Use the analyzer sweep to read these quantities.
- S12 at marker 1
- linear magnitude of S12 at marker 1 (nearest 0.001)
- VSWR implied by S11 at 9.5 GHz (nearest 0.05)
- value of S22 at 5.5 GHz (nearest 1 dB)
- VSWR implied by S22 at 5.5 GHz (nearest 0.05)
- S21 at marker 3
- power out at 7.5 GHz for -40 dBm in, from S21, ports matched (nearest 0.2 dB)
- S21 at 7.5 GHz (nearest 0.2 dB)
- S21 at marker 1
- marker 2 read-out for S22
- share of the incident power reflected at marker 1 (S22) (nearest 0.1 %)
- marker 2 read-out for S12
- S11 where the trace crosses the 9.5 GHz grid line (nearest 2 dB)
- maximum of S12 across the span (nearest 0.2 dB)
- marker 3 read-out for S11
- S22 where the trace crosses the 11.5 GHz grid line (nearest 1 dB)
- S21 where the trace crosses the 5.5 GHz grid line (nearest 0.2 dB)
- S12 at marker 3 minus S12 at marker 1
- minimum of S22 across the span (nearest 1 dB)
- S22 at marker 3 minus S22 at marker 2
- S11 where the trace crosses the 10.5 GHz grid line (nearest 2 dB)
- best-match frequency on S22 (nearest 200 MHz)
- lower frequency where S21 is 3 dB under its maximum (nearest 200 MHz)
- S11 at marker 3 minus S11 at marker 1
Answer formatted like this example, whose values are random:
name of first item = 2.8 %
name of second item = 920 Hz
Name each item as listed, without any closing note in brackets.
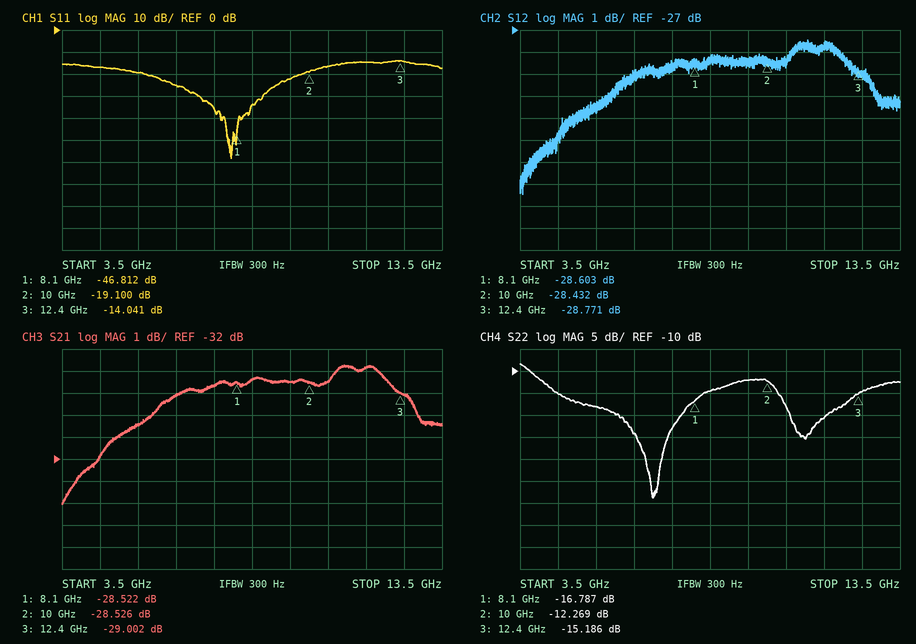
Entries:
S12 at marker 1 = -28.603 dB
linear magnitude of S12 at marker 1 = 0.037
VSWR implied by S11 at 9.5 GHz = 1.15
value of S22 at 5.5 GHz = -18 dB
VSWR implied by S22 at 5.5 GHz = 1.30
S21 at marker 3 = -29.002 dB
power out at 7.5 GHz for -40 dBm in, from S21, ports matched = -68.6 dBm
S21 at 7.5 GHz = -28.6 dB
S21 at marker 1 = -28.522 dB
marker 2 read-out for S22 = -12.269 dB
share of the incident power reflected at marker 1 (S22) = 2.1 %
marker 2 read-out for S12 = -28.432 dB
S11 where the trace crosses the 9.5 GHz grid line = -22 dB
maximum of S12 across the span = -27.4 dB
marker 3 read-out for S11 = -14.041 dB
S22 where the trace crosses the 11.5 GHz grid line = -21 dB
S21 where the trace crosses the 5.5 GHz grid line = -30.4 dB
S12 at marker 3 minus S12 at marker 1 = -0.168 dB
minimum of S22 across the span = -39 dB
S22 at marker 3 minus S22 at marker 2 = -2.917 dB
S11 where the trace crosses the 10.5 GHz grid line = -16 dB
best-match frequency on S22 = 7.0 GHz
lower frequency where S21 is 3 dB under its maximum = 5.2 GHz
S11 at marker 3 minus S11 at marker 1 = 32.771 dB
